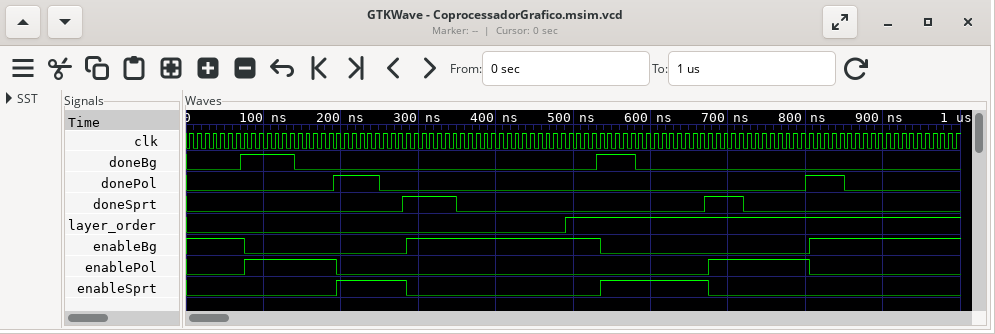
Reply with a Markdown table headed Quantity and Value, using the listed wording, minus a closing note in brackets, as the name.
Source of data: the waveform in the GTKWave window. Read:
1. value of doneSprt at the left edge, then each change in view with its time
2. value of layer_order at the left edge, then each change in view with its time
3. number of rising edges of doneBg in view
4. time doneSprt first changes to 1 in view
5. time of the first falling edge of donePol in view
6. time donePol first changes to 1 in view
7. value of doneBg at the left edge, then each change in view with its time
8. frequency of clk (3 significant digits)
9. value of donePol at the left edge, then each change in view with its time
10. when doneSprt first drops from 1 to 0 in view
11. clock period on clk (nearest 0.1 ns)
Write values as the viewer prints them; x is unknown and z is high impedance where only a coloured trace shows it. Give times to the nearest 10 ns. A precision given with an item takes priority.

| Quantity | Value |
|---|---|
| value of doneSprt at the left edge, then each change in view with its time | 0, 1 at 280 ns, 0 at 350 ns, 1 at 670 ns, 0 at 720 ns |
| value of layer_order at the left edge, then each change in view with its time | 0, 1 at 490 ns |
| number of rising edges of doneBg in view | 2 |
| time doneSprt first changes to 1 in view | 280 ns |
| time of the first falling edge of donePol in view | 250 ns |
| time donePol first changes to 1 in view | 190 ns |
| value of doneBg at the left edge, then each change in view with its time | 0, 1 at 70 ns, 0 at 140 ns, 1 at 530 ns, 0 at 580 ns |
| frequency of clk | 100 MHz |
| value of donePol at the left edge, then each change in view with its time | 0, 1 at 190 ns, 0 at 250 ns, 1 at 800 ns, 0 at 850 ns |
| when doneSprt first drops from 1 to 0 in view | 350 ns |
| clock period on clk | 10 ns |
